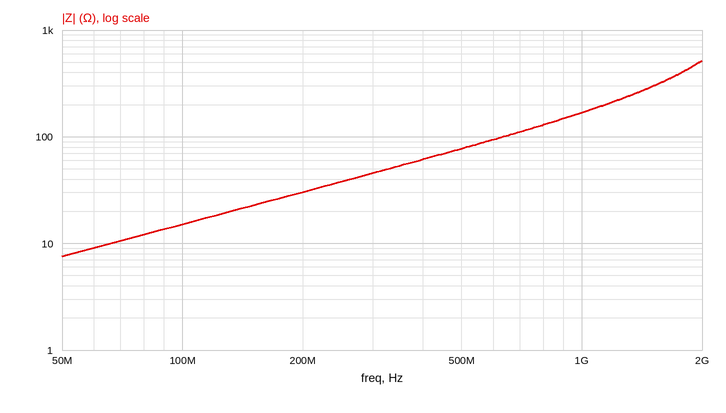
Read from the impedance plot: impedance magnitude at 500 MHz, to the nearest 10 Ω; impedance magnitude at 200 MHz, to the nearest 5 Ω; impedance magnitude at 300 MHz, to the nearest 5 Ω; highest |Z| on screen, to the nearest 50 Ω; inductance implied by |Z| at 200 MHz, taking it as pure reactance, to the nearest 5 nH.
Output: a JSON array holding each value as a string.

["80 Ω", "30 Ω", "45 Ω", "500 Ω", "25 nH"]
